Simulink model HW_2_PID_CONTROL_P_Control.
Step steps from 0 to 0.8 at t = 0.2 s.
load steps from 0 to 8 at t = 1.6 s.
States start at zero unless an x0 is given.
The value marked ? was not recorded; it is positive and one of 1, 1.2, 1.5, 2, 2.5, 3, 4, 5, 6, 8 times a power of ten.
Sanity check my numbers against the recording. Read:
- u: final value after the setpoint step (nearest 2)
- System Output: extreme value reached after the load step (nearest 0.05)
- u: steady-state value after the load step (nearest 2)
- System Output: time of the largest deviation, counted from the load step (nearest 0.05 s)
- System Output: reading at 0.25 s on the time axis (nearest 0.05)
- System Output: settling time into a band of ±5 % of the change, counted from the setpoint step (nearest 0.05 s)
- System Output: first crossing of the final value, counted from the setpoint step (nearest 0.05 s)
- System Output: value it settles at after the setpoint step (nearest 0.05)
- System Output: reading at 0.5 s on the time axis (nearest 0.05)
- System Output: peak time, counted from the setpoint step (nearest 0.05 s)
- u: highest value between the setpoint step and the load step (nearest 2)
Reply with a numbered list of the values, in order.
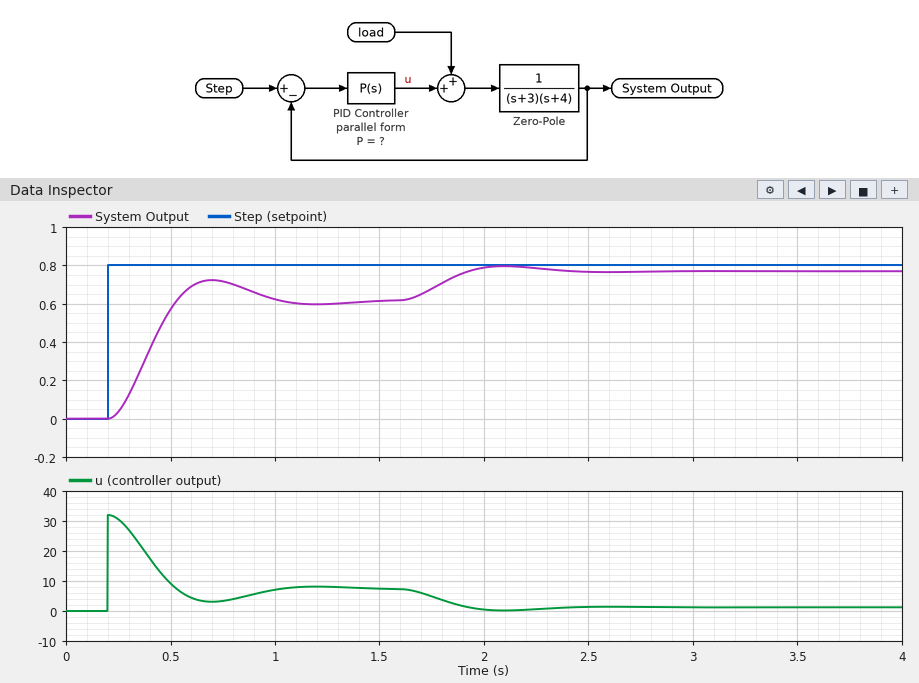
1. 8
2. 0.80
3. 2
4. 0.50 s
5. 0.05
6. 0.75 s
7. 0.35 s
8. 0.60
9. 0.55
10. 0.50 s
11. 32
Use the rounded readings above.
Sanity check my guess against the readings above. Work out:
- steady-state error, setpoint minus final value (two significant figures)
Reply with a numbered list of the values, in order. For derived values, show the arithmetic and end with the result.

1. 0.8 - 0.6 = 0.20
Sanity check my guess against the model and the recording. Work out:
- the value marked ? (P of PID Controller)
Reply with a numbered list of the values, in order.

1. 40
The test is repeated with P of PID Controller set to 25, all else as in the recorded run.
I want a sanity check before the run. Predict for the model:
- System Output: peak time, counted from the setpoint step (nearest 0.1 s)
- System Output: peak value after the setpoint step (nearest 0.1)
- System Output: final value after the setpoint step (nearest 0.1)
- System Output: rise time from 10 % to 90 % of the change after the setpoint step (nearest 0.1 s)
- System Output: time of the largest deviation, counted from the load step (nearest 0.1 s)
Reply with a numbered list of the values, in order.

1. 0.6 s
2. 0.6
3. 0.5
4. 0.3 s
5. 0.6 s
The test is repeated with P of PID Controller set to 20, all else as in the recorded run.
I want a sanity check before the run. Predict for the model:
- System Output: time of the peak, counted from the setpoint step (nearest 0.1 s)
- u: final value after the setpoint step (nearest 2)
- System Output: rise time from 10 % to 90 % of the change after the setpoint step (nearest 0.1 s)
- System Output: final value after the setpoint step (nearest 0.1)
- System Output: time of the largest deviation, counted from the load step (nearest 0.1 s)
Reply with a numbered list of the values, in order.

1. 0.7 s
2. 6
3. 0.3 s
4. 0.5
5. 0.7 s
